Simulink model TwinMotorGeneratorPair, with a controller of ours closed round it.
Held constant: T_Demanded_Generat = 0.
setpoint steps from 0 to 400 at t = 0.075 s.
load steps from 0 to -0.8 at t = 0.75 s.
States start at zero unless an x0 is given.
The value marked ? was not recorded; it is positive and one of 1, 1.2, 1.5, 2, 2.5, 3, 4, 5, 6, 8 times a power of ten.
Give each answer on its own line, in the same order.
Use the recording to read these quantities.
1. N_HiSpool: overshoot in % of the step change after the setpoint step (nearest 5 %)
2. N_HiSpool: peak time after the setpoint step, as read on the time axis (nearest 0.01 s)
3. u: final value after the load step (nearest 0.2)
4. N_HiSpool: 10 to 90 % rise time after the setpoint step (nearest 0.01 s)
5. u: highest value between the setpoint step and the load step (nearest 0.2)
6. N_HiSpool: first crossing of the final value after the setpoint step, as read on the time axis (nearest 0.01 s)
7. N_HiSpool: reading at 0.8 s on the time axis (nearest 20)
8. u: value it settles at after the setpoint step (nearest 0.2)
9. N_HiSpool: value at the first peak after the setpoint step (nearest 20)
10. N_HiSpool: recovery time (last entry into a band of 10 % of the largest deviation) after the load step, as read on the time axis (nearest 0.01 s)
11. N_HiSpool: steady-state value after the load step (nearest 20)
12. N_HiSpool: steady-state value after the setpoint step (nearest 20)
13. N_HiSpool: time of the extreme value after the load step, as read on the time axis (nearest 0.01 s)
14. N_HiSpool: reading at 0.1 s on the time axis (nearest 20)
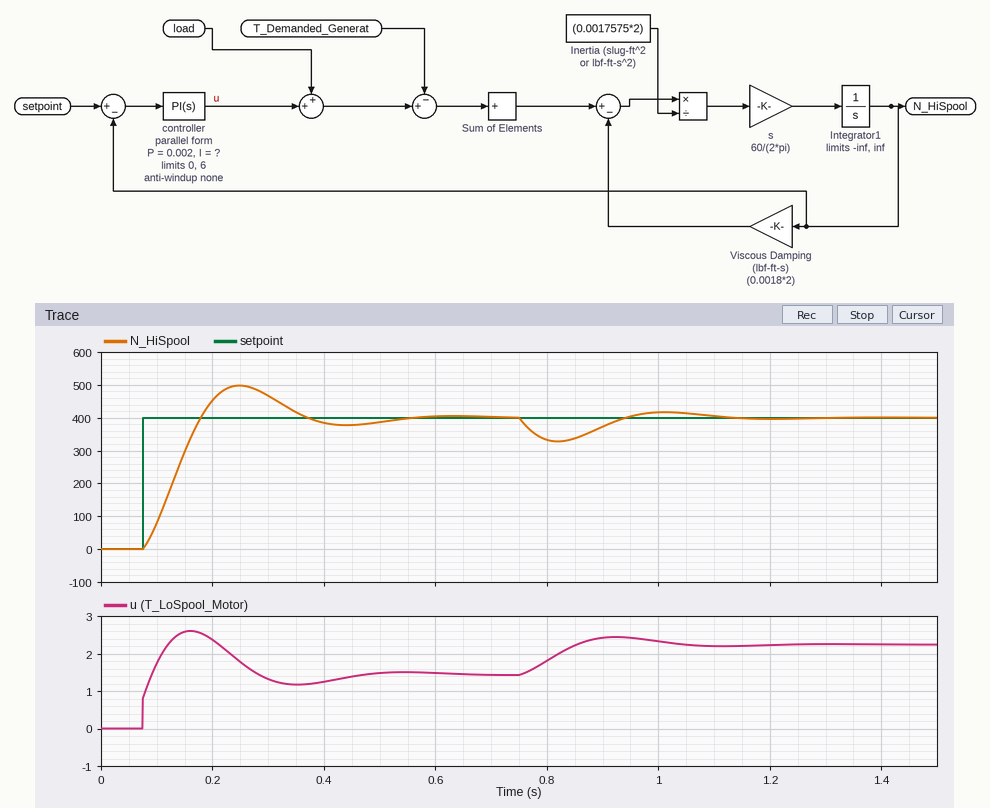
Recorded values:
25 %
0.25 s
2.2
0.08 s
2.6
0.18 s
340
1.4
500
1.09 s
400
400
0.82 s
80
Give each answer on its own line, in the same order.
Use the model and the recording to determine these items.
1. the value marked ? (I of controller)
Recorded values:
0.12
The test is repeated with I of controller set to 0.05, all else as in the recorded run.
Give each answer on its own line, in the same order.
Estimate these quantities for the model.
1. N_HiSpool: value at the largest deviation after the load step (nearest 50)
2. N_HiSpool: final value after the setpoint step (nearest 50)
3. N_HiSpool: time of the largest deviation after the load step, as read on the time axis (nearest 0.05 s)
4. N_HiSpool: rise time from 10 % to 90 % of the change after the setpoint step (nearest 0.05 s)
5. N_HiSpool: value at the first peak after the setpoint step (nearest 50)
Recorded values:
300
400
0.85 s
0.15 s
450
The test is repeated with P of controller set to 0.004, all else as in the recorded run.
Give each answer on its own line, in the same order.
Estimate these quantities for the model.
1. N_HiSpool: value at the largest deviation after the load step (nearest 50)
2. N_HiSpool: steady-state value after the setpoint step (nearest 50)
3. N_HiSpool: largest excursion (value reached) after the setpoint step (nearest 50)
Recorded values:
350
400
450
